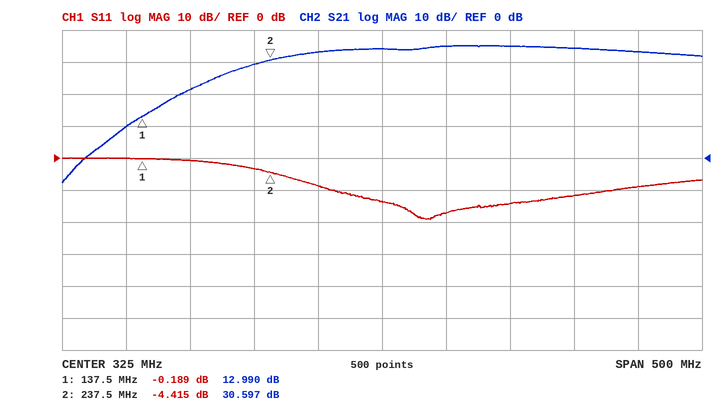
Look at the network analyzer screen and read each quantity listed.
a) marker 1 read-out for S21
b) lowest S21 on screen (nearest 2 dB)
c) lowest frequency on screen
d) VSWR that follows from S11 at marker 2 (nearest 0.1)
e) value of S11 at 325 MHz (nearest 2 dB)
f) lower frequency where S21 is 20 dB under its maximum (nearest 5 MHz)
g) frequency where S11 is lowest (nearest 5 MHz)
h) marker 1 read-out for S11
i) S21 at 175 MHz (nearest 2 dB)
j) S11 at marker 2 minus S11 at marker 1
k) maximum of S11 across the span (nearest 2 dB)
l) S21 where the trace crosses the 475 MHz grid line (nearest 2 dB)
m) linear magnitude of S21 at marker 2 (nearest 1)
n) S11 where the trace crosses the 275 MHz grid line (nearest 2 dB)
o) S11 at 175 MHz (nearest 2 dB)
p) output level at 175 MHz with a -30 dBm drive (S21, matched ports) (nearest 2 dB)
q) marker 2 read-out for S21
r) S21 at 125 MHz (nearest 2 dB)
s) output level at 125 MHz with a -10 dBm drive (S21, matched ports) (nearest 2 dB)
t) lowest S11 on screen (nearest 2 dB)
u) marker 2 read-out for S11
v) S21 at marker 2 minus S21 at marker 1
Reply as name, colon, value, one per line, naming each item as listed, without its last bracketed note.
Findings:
marker 1 read-out for S21: 12.990 dB
lowest S21 on screen: -8 dB
lowest frequency on screen: 75 MHz
VSWR that follows from S11 at marker 2: 4.0
value of S11 at 325 MHz: -14 dB
lower frequency where S21 is 20 dB under its maximum: 145 MHz
frequency where S11 is lowest: 360 MHz
marker 1 read-out for S11: -0.189 dB
S21 at 175 MHz: 22 dB
S11 at marker 2 minus S11 at marker 1: -4.226 dB
maximum of S11 across the span: 0 dB
S21 where the trace crosses the 475 MHz grid line: 34 dB
linear magnitude of S21 at marker 2: 34
S11 where the trace crosses the 275 MHz grid line: -8 dB
S11 at 175 MHz: 0 dB
output level at 175 MHz with a -30 dBm drive (S21, matched ports): -8 dBm
marker 2 read-out for S21: 30.597 dB
S21 at 125 MHz: 10 dB
output level at 125 MHz with a -10 dBm drive (S21, matched ports): 0 dBm
lowest S11 on screen: -20 dB
marker 2 read-out for S11: -4.415 dB
S21 at marker 2 minus S21 at marker 1: 17.607 dB
